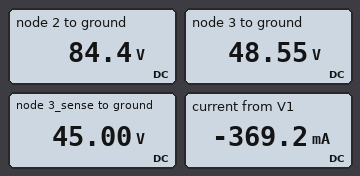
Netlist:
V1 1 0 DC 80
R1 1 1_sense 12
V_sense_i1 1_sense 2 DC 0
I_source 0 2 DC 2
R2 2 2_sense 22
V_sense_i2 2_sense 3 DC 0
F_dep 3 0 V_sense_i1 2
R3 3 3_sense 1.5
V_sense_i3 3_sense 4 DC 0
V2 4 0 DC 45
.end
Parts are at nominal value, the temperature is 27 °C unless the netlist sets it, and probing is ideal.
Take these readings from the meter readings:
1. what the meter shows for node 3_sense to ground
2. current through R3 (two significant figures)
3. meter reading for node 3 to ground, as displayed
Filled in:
45.00 V
2.4 A
48.55 V
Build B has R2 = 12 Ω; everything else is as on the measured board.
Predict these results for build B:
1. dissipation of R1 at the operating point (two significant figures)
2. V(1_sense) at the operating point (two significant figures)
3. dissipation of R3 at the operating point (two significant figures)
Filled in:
1.5 W
76 V
4.1 W
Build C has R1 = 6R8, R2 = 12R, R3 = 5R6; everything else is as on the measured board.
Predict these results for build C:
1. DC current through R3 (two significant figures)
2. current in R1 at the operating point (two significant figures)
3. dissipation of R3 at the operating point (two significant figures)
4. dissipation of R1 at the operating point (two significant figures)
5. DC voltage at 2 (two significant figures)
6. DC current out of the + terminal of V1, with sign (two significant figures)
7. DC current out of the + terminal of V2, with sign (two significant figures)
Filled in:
2.0 A
15 mA
23 W
1.6 mW
80 V
-15 mA
-2.0 A
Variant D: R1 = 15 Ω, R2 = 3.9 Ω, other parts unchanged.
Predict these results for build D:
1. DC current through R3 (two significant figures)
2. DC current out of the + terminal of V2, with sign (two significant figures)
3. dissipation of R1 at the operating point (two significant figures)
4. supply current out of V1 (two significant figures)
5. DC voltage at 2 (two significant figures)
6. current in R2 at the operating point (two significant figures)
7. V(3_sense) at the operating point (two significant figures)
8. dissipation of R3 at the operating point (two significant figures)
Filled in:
610 mA
-610 mA
29 W
1.4 A
59 V
3.4 A
45 V
560 mW
